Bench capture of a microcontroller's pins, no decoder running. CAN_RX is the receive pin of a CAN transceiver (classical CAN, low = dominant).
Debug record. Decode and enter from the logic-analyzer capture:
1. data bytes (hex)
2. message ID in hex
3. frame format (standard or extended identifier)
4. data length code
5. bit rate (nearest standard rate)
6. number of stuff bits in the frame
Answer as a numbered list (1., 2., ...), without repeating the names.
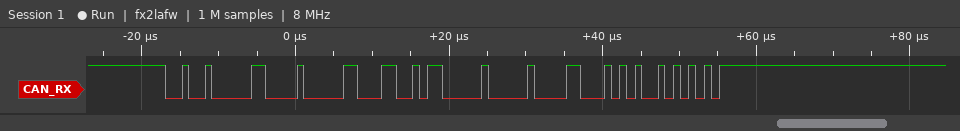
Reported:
1. 11 96 00 06
2. 0x241
3. standard
4. 4
5. 1000 kbit/s
6. 4
